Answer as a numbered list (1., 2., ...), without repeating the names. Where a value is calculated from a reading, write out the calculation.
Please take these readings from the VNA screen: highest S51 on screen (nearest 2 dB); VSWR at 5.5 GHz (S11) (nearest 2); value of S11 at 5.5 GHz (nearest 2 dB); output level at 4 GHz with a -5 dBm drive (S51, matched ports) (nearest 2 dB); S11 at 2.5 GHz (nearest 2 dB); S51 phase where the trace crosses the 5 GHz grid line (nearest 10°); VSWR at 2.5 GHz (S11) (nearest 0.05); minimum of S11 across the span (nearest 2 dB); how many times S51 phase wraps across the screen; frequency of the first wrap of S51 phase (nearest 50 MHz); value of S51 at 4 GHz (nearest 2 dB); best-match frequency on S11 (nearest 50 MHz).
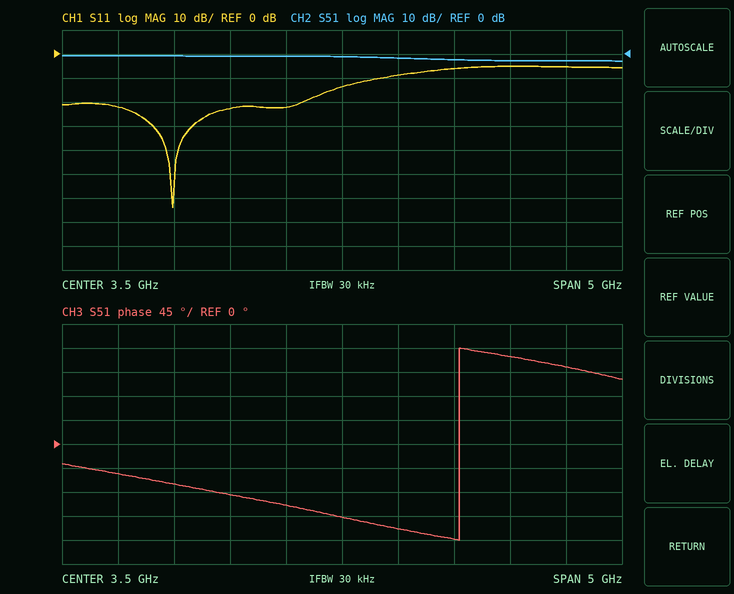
1. 0 dB
2. |Γ| = 10^(-6/20) = 0.5012; VSWR = (1 + 0.5012)/(1 − 0.5012) ≈ 3.01, so 4 to the nearest 2
3. -6 dB
4. -5 dBm + (-2 dB) = -6 dBm
5. -22 dB
6. 160°
7. |Γ| = 10^(-22/20) = 0.0794; VSWR = (1 + 0.0794)/(1 − 0.0794) ≈ 1.17, so 1.15 to the nearest 0.05
8. -64 dB
9. 1
10. 4.55 GHz
11. -2 dB
12. 2.00 GHz
